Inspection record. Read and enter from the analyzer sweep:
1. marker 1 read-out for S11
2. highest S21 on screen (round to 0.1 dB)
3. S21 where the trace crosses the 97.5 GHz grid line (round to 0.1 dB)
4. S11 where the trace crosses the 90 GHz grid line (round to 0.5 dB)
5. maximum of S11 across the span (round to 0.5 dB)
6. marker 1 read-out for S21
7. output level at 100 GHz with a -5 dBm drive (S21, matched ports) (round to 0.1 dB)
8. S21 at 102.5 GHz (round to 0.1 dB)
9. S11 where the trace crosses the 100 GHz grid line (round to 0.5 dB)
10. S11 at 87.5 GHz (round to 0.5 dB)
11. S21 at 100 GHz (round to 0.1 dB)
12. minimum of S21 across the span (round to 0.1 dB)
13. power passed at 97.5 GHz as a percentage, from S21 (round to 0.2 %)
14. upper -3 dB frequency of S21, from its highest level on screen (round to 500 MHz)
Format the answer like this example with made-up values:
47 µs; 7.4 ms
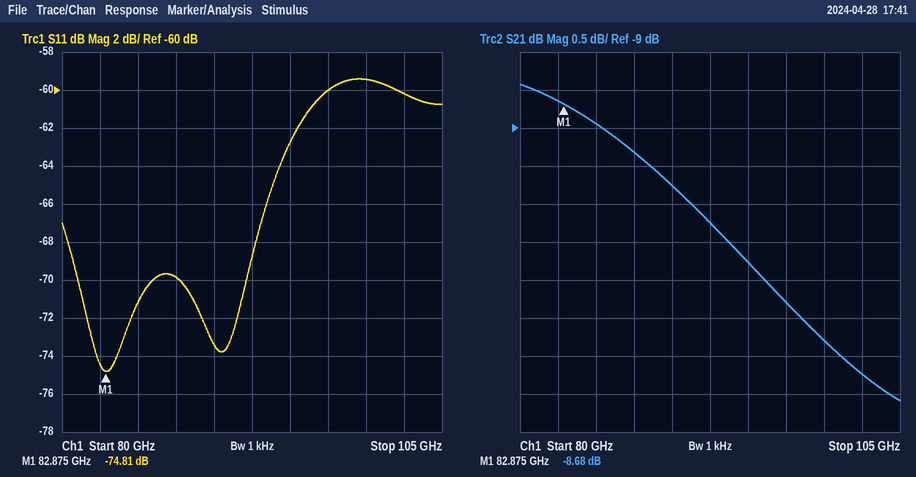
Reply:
-74.81 dB; -8.4 dB; -11.3 dB; -73.5 dB; -59.5 dB; -8.68 dB; -16.8 dBm; -12.2 dB; -59.5 dB; -70.0 dB; -11.8 dB; -12.6 dB; 7.4 %; 98.0 GHz
